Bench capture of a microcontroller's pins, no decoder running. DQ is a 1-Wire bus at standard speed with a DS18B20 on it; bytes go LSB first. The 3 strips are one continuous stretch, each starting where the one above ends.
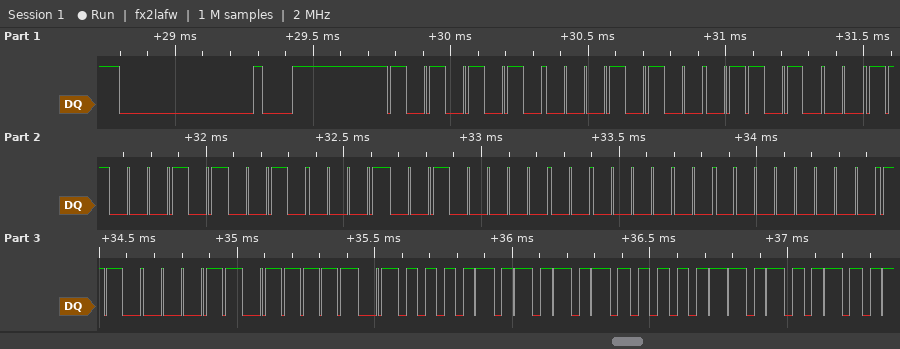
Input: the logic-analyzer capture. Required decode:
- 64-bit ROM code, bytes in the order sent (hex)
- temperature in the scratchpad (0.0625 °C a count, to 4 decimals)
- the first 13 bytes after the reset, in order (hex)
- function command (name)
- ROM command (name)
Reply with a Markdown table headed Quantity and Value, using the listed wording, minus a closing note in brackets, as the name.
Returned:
| Quantity | Value |
|---|---|
| 64-bit ROM code, bytes in the order sent | 28 16 A3 84 04 00 00 C3 |
| temperature in the scratchpad | 85.0000 °C |
| the first 13 bytes after the reset, in order | 55 28 16 A3 84 04 00 00 C3 BE 50 05 4B |
| function command | Read Scratchpad |
| ROM command | Match ROM |
